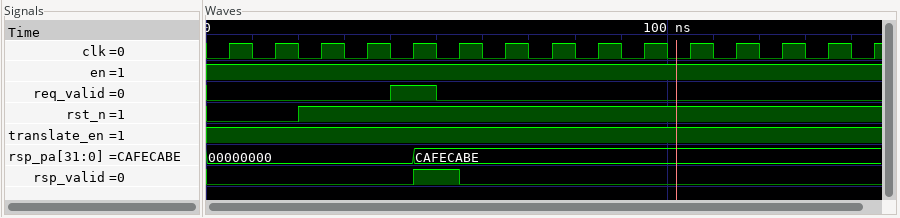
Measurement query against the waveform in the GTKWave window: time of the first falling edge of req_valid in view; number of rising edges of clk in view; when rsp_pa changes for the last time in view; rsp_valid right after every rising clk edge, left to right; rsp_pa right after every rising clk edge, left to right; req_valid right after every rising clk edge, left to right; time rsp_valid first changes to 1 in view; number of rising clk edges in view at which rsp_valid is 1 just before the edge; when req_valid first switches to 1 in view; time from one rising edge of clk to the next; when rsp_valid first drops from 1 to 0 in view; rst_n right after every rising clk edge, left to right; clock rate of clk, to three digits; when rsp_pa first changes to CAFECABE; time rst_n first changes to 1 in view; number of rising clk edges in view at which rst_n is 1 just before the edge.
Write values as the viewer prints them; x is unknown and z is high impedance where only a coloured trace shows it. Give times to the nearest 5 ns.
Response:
50 ns
15
45 ns
0 0 0 0 1 0 0 0 0 0 0 0 0 0 0
00000000, 00000000, 00000000, 00000000, CAFECABE, CAFECABE, CAFECABE, CAFECABE, CAFECABE, CAFECABE, CAFECABE, CAFECABE, CAFECABE, CAFECABE, CAFECABE
0 0 0 0 1 0 0 0 0 0 0 0 0 0 0
45 ns
1
40 ns
10 ns
55 ns
0 0 1 1 1 1 1 1 1 1 1 1 1 1 1
100 MHz
45 ns
20 ns
13
